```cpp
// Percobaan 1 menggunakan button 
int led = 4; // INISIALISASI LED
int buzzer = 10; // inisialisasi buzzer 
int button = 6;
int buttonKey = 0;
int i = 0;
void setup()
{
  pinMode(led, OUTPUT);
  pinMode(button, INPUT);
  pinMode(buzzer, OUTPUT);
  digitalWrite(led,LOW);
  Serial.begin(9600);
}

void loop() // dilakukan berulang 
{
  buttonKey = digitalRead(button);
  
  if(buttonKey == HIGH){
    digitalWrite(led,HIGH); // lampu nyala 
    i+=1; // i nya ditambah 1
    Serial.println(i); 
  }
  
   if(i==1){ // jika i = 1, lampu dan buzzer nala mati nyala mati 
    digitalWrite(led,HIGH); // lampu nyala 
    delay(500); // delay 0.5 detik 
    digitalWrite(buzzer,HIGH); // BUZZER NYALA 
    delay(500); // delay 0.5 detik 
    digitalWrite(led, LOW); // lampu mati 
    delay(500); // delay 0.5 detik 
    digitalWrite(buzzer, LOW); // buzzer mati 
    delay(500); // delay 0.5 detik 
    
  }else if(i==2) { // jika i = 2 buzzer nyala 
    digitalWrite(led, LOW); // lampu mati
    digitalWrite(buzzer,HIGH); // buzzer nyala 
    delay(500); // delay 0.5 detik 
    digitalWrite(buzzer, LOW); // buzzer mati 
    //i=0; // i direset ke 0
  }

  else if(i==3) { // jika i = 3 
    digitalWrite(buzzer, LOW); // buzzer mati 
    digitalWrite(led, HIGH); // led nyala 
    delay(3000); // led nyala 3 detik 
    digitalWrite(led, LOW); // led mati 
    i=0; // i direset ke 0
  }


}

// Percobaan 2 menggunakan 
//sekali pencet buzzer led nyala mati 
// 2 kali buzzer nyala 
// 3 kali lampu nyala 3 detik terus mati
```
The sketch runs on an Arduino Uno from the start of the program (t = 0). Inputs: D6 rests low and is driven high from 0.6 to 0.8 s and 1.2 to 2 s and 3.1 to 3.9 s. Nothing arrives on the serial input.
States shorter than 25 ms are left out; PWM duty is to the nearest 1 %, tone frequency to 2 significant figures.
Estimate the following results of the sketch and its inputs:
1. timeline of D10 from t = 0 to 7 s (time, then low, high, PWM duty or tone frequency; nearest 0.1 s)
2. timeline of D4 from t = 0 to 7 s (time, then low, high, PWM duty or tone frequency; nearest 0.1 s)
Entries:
0 s low; 1.1 s high; 2.1 s low; 3.1 s high; 4.1 s low; 5.1 s high; 6.1 s low
0 s low; 0.6 s high; 1.6 s low; 2.6 s high; 3.6 s low; 4.6 s high; 5.6 s low; 6.6 s high
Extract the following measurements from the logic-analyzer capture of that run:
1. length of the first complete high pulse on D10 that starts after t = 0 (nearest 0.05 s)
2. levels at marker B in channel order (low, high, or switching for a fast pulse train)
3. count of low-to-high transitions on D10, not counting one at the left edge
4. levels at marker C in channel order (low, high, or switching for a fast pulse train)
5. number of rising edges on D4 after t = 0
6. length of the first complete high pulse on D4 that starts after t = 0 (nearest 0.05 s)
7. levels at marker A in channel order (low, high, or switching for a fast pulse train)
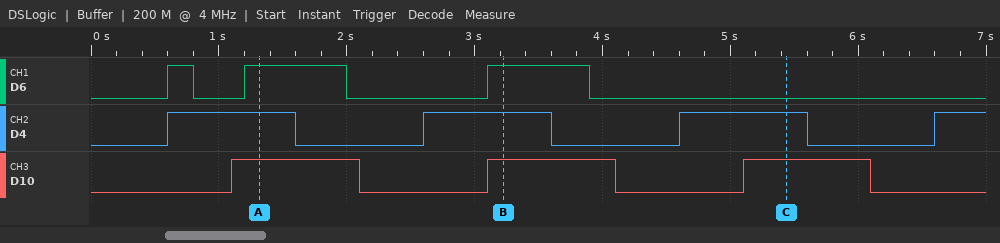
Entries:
1.00 s
D6 high, D4 high, D10 high
3
D6 low, D4 high, D10 high
4
1.00 s
D6 high, D4 high, D10 high
